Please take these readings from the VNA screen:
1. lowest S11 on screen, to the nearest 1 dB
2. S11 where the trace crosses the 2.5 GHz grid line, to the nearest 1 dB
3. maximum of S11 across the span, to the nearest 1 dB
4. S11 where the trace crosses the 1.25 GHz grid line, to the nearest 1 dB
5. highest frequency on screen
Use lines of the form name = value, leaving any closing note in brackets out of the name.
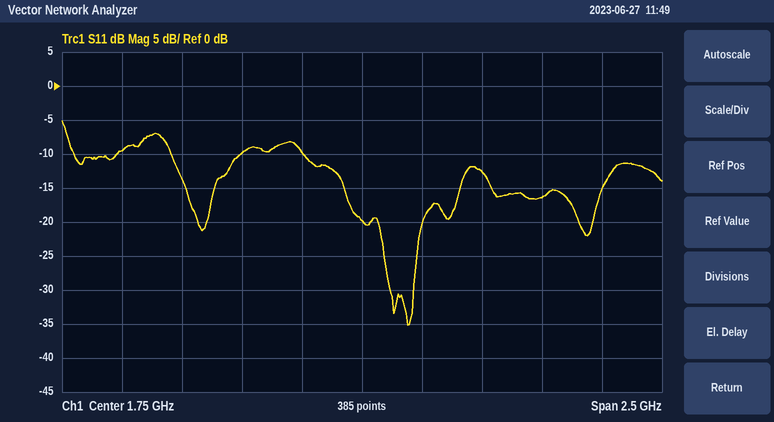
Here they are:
lowest S11 on screen, to the nearest 1 dB = -35 dB
S11 where the trace crosses the 2.5 GHz grid line, to the nearest 1 dB = -16 dB
maximum of S11 across the span, to the nearest 1 dB = -5 dB
S11 where the trace crosses the 1.25 GHz grid line, to the nearest 1 dB = -10 dB
highest frequency on screen = 3 GHz
